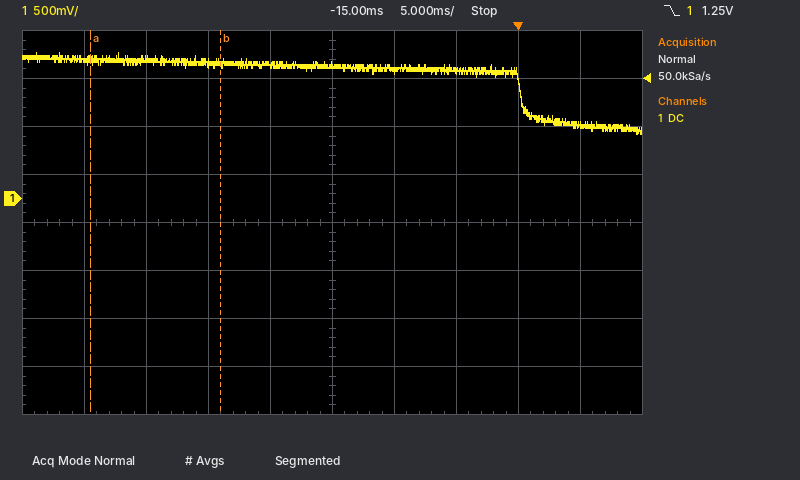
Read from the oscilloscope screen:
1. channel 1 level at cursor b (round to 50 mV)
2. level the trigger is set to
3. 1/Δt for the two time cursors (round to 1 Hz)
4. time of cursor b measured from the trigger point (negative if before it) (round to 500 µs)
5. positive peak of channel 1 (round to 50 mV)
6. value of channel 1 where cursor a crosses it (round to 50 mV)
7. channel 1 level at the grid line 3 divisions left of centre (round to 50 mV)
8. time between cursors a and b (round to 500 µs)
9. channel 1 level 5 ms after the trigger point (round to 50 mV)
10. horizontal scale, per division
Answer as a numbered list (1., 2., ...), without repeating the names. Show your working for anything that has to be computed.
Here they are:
1. 1.40 V
2. 1.25 V
3. 1 / 10.5 ms ≈ 95 Hz
4. -24.0 ms
5. 1.50 V
6. 1.45 V
7. 1.45 V
8. 10.5 ms
9. 750 mV
10. 5 ms
